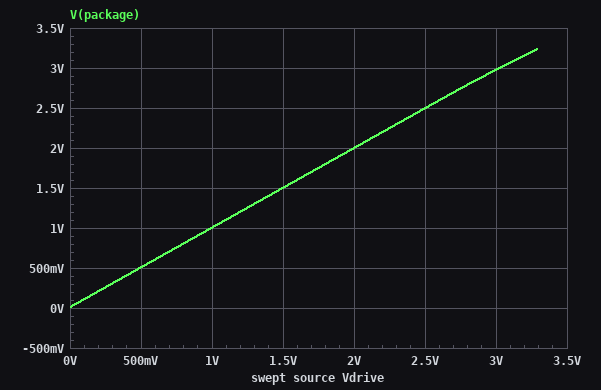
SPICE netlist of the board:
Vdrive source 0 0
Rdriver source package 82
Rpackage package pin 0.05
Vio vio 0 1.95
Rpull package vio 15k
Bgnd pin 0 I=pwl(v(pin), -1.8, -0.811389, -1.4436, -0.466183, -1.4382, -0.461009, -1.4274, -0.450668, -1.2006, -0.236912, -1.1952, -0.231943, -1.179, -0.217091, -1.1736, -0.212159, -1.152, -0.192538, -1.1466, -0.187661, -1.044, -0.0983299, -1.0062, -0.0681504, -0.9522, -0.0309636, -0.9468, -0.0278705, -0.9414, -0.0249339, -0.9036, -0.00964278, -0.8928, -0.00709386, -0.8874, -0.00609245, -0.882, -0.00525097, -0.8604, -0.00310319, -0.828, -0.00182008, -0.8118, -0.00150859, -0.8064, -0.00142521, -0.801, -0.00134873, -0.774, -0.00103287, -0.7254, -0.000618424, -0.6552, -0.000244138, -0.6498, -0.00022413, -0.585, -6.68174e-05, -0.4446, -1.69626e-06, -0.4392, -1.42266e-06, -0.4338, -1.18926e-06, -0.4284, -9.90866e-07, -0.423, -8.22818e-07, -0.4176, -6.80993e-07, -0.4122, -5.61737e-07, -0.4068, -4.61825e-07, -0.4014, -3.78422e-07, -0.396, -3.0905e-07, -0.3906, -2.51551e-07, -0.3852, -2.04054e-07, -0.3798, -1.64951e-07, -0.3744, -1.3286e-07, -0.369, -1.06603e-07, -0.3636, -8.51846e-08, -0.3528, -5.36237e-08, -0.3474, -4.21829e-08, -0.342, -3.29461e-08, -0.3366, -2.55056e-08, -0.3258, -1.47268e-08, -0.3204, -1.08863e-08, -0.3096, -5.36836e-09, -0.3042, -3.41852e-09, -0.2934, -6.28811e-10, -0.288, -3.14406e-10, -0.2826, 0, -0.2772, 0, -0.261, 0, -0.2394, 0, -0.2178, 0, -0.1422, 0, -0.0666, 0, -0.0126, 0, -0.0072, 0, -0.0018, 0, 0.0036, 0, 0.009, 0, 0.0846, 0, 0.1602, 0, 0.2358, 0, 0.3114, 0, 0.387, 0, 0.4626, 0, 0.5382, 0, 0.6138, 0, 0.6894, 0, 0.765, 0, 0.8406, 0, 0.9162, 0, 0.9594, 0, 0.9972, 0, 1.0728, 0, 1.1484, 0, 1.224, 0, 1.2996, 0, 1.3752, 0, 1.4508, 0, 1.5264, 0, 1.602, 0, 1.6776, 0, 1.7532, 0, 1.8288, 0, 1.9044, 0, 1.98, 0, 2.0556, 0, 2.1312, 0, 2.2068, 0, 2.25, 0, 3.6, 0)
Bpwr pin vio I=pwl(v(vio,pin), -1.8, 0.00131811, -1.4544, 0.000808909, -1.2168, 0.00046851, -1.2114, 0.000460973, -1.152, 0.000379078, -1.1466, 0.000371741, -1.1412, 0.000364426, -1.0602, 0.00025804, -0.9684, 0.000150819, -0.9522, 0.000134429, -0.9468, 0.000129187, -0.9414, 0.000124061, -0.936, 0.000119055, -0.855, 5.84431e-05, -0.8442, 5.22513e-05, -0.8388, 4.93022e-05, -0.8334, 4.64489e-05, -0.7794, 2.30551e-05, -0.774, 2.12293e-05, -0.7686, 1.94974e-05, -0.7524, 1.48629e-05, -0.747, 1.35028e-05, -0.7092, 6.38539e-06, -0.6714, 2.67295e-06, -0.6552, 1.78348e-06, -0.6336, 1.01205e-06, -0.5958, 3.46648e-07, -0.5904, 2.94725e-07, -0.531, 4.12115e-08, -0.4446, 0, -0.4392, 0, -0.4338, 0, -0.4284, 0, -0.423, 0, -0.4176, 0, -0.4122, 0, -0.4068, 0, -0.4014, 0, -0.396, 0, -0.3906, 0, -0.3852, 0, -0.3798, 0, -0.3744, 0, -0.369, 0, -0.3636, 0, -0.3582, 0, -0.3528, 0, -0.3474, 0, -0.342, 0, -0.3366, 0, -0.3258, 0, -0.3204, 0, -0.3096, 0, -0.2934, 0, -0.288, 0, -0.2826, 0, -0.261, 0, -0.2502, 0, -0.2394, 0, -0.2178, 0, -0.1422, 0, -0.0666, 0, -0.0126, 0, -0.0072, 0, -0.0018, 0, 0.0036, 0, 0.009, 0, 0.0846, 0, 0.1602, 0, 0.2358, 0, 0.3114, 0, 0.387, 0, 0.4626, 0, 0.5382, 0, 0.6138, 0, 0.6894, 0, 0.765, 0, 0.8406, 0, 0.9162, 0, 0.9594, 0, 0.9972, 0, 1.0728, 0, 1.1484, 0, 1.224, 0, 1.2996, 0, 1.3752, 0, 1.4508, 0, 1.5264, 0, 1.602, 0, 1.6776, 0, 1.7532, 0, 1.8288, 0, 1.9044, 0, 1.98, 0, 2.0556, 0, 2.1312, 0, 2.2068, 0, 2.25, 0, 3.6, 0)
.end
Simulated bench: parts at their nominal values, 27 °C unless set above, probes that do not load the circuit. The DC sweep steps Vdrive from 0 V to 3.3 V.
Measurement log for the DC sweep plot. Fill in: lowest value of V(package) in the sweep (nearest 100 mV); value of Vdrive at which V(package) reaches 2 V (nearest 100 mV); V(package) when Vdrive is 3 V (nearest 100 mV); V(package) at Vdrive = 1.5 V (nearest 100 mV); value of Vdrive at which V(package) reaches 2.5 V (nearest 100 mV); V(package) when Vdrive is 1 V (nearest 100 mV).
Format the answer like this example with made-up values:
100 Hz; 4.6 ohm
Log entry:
0 V; 2.0 V; 3.0 V; 1.5 V; 2.5 V; 1.0 V
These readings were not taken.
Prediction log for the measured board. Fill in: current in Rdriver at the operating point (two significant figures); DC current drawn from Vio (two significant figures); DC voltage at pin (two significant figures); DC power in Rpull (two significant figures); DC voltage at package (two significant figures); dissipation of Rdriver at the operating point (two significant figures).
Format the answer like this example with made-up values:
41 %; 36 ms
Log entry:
130 µA; 130 µA; 11 mV; 250 µW; 11 mV; 1.4 µW
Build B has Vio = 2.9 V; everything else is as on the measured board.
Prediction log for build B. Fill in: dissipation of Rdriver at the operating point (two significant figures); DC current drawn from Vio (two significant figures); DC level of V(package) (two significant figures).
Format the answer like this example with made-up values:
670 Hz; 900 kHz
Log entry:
3.0 µW; 190 µA; 16 mV
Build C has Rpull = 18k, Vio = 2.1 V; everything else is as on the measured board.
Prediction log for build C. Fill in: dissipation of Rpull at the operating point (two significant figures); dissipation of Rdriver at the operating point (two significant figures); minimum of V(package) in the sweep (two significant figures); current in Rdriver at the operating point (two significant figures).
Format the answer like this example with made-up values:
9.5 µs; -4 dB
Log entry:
240 µW; 1.1 µW; 9.5 mV; 120 µA
